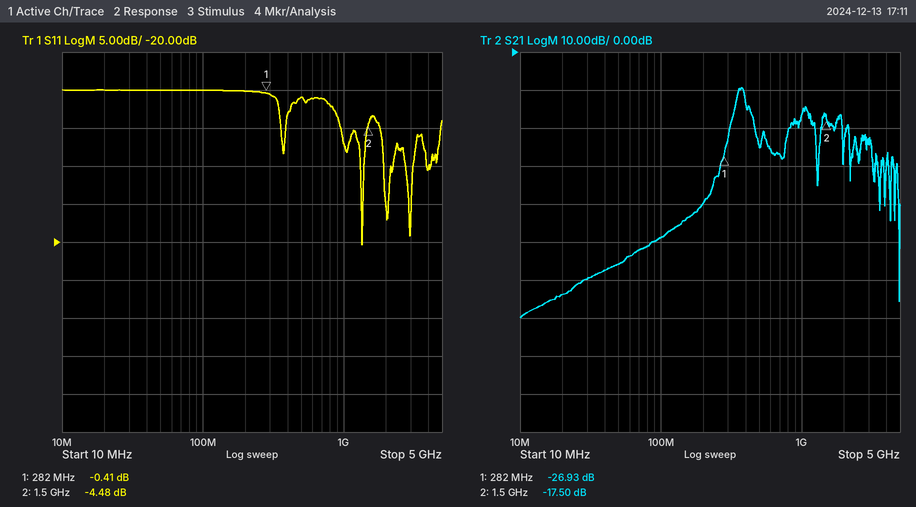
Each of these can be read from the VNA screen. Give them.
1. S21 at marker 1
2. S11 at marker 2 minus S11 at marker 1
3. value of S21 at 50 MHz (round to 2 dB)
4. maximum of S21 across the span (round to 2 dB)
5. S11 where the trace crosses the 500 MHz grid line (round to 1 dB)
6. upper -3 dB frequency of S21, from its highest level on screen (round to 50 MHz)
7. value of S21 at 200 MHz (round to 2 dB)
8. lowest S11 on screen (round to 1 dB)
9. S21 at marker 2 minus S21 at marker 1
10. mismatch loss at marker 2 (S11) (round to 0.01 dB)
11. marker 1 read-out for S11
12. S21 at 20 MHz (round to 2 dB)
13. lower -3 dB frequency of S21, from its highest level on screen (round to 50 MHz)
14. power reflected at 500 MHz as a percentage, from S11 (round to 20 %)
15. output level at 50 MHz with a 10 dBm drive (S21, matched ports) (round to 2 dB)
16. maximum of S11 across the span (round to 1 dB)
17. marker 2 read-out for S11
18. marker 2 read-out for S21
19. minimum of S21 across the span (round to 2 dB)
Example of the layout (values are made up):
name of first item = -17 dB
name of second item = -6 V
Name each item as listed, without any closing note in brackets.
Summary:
S21 at marker 1 = -26.93 dB
S11 at marker 2 minus S11 at marker 1 = -4.07 dB
value of S21 at 50 MHz = -56 dB
maximum of S21 across the span = -10 dB
S11 where the trace crosses the 500 MHz grid line = -1 dB
upper -3 dB frequency of S21, from its highest level on screen = 400 MHz
value of S21 at 200 MHz = -40 dB
lowest S11 on screen = -20 dB
S21 at marker 2 minus S21 at marker 1 = 9.43 dB
mismatch loss at marker 2 (S11) = 1.91 dB
marker 1 read-out for S11 = -0.41 dB
S21 at 20 MHz = -64 dB
lower -3 dB frequency of S21, from its highest level on screen = 350 MHz
power reflected at 500 MHz as a percentage, from S11 = 80 %
output level at 50 MHz with a 10 dBm drive (S21, matched ports) = -46 dBm
maximum of S11 across the span = 0 dB
marker 2 read-out for S11 = -4.48 dB
marker 2 read-out for S21 = -17.50 dB
minimum of S21 across the span = -70 dB
